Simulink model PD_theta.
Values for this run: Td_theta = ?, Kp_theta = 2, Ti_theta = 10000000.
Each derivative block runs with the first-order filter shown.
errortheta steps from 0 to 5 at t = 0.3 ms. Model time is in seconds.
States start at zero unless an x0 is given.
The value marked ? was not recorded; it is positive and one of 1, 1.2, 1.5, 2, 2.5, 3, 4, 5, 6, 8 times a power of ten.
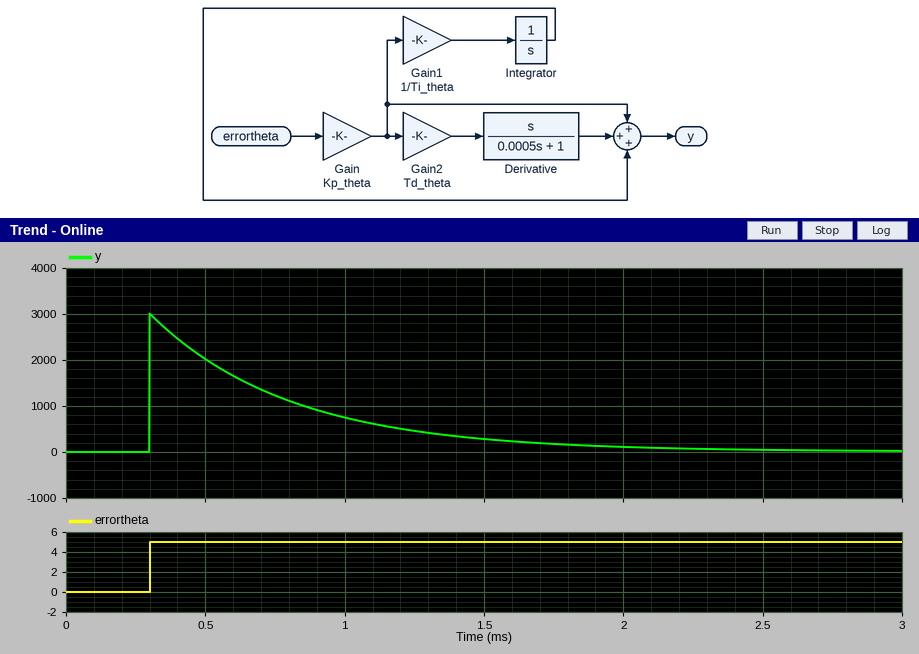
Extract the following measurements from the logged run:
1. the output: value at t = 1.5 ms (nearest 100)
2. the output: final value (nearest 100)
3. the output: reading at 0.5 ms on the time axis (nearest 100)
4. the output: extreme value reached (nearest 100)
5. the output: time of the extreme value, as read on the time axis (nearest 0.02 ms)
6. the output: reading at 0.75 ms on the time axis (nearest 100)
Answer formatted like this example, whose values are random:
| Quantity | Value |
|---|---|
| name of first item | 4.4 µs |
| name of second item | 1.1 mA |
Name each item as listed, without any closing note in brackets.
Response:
| Quantity | Value |
|---|---|
| the output: value at t = 1.5 ms | 300 |
| the output: final value | 0 |
| the output: reading at 0.5 ms on the time axis | 2000 |
| the output: extreme value reached | 3000 |
| the output: time of the extreme value, as read on the time axis | 0.30 ms |
| the output: reading at 0.75 ms on the time axis | 1200 |
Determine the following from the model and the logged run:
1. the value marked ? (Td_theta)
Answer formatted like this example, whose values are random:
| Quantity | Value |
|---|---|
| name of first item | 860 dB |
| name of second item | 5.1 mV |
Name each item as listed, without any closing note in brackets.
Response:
| Quantity | Value |
|---|---|
| the value marked ? | 0.15 |
